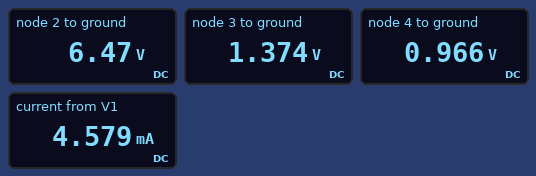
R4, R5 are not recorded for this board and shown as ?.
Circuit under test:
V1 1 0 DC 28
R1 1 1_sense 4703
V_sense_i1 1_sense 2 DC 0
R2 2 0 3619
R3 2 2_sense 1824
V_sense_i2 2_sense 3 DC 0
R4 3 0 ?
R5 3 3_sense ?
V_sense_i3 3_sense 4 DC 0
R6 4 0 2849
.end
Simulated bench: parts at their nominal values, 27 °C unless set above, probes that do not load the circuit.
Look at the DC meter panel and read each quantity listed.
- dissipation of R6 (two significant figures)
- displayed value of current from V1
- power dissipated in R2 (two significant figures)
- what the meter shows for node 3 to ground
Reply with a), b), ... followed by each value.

a) 330 µW
b) 4.579 mA
c) 12 mW
d) 1.374 V
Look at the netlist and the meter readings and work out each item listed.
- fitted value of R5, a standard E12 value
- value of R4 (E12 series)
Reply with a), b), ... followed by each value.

a) 1.2 kΩ
b) 560 Ω
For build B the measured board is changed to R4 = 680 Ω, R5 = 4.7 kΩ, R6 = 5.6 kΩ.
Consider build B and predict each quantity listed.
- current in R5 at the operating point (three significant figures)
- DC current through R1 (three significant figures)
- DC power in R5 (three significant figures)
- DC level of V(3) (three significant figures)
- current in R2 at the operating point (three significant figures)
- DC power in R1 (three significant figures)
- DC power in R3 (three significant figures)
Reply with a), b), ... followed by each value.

a) 167 µA
b) 4.54 mA
c) 132 µW
d) 1.72 V
e) 1.84 mA
f) 96.9 mW
g) 13.3 mW
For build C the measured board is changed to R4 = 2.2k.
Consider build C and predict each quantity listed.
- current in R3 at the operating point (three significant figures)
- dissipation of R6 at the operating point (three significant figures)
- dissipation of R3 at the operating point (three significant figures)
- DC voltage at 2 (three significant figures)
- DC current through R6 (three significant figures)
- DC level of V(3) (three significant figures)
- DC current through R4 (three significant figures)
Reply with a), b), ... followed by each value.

a) 2.30 mA
b) 1.87 mW
c) 9.65 mW
d) 7.47 V
e) 810 µA
f) 3.28 V
g) 1.49 mA
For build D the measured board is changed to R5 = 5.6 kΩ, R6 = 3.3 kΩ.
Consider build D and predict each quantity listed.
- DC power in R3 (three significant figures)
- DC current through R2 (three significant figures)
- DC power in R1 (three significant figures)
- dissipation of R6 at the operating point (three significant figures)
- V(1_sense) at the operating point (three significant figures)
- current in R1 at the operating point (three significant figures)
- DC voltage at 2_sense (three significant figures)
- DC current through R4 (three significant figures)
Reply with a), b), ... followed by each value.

a) 14.0 mW
b) 1.80 mA
c) 98.2 mW
d) 88.7 µW
e) 6.51 V
f) 4.57 mA
g) 1.46 V
h) 2.61 mA
